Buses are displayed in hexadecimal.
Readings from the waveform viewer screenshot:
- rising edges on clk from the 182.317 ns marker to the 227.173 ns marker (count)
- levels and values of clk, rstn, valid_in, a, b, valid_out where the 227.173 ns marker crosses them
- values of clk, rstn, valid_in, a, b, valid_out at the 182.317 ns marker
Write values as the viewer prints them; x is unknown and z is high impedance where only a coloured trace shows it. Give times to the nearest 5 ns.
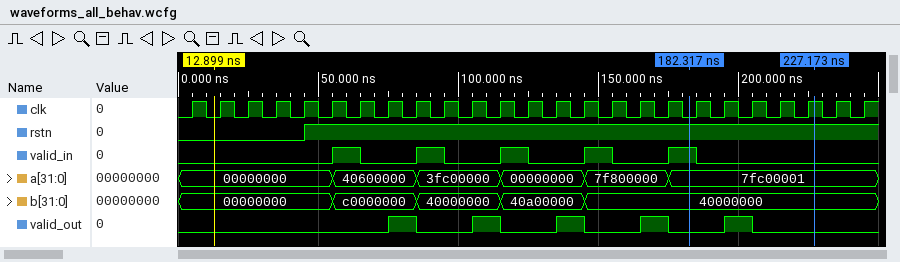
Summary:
5
clk=1, rstn=1, valid_in=0, a=7fc00001, b=40000000, valid_out=0
clk=0, rstn=1, valid_in=1, a=7fc00001, b=40000000, valid_out=0
